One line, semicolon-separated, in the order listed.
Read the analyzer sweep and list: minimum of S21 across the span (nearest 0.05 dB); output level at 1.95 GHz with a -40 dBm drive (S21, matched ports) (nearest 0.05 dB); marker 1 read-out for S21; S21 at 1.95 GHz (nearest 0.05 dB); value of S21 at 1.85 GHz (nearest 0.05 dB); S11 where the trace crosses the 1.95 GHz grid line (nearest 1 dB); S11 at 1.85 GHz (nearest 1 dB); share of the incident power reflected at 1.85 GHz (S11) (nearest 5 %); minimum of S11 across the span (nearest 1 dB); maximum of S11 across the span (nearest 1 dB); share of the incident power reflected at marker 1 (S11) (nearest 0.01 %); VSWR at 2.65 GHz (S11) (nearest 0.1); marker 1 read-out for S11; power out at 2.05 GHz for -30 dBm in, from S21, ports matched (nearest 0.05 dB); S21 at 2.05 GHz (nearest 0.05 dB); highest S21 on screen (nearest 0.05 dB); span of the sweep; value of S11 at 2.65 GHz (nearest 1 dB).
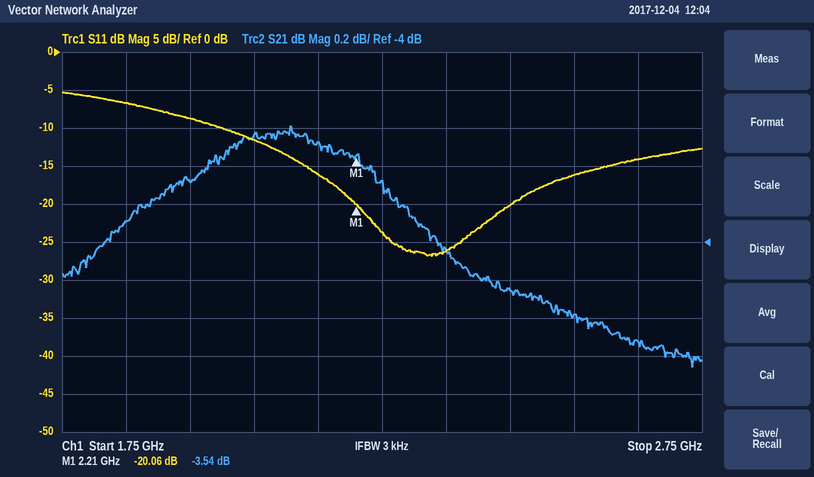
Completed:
-4.65 dB; -43.70 dBm; -3.54 dB; -3.70 dB; -3.90 dB; -9 dB; -7 dB; 20 %; -27 dB; -5 dB; 0.99 %; 1.5; -20.06 dB; -33.45 dBm; -3.45 dB; -3.40 dB; 1 GHz; -14 dB
